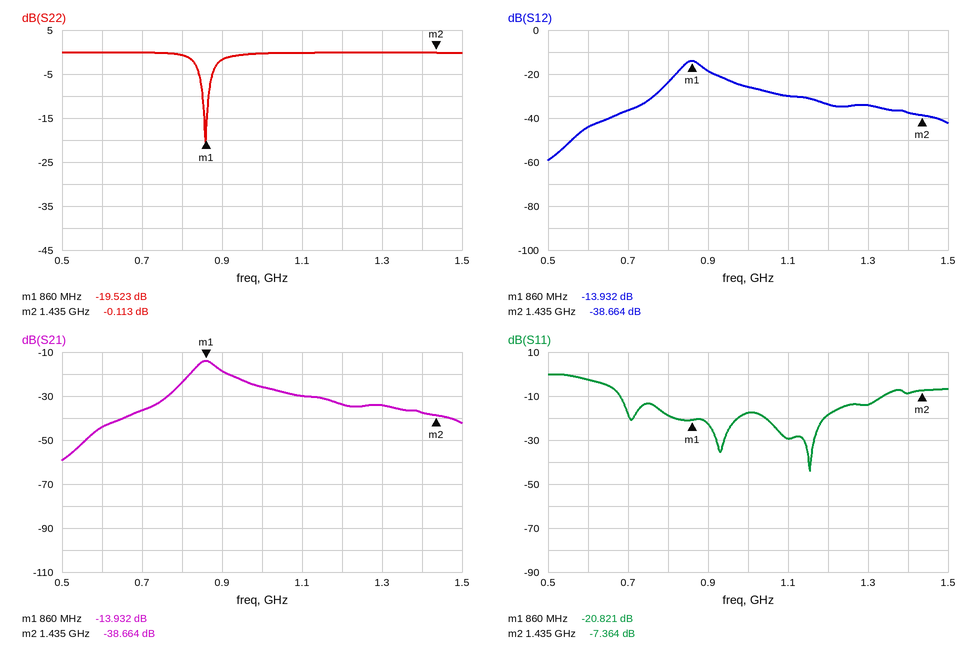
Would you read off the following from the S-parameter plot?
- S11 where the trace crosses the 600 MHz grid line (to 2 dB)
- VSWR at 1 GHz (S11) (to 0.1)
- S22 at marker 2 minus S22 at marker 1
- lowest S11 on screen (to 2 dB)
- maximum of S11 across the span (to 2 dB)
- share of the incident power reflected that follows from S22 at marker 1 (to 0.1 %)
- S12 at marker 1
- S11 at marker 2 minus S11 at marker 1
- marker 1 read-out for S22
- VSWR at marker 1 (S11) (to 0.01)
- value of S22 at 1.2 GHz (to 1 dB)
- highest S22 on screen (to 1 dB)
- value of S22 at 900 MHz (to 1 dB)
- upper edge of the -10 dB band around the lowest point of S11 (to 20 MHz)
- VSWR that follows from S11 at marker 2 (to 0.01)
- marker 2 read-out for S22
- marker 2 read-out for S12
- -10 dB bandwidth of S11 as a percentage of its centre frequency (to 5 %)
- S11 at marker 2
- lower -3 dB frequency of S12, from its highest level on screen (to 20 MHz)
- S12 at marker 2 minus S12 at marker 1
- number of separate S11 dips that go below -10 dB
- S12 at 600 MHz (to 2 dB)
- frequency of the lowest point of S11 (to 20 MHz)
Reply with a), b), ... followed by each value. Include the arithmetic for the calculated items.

a) -2 dB
b) |Γ| = 10^(-18/20) = 0.1259; VSWR = (1 + 0.1259)/(1 − 0.1259) ≈ 1.3
c) -0.113 − (-19.523) = 19.410 dB
d) -44 dB
e) 0 dB
f) 10^(-19.523/10) ≈ 1.1 %
g) -13.932 dB
h) -7.364 − (-20.821) = 13.457 dB
i) -19.523 dB
j) (1 + 0.0910)/(1 − 0.0910) ≈ 1.20
k) 0 dB
l) 0 dB
m) -2 dB
n) 1.34 GHz
o) (1 + 0.4284)/(1 − 0.4284) ≈ 2.50
p) -0.113 dB
q) -38.664 dB
r) 660 MHz / 1.01 GHz ≈ 65 %
s) -7.364 dB
t) 840 MHz
u) -38.664 − (-13.932) = -24.732 dB
v) 3
w) -44 dB
x) 1.16 GHz
